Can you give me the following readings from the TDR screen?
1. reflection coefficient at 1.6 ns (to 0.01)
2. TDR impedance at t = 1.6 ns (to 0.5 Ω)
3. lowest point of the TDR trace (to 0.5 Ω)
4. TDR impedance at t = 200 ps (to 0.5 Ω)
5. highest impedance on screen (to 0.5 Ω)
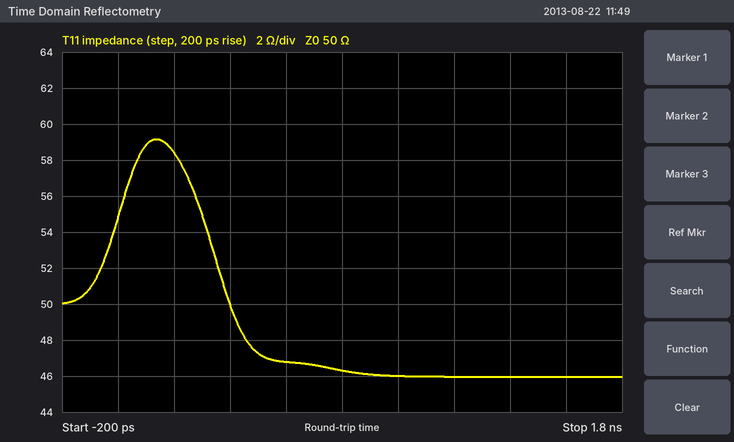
-0.04
46.0 Ω
46.0 Ω
58.5 Ω
59.0 Ω
